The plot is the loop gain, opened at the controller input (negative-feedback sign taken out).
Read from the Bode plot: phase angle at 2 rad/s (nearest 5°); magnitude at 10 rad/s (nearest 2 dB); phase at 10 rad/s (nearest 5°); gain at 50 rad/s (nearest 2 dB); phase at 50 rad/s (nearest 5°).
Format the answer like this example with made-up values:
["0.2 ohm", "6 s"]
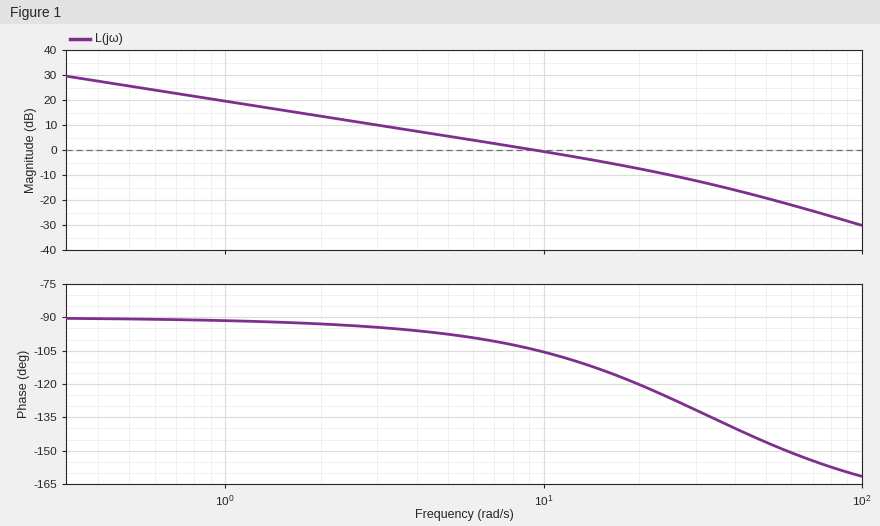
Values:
["-95°", "0 dB", "-105°", "-20 dB", "-145°"]
